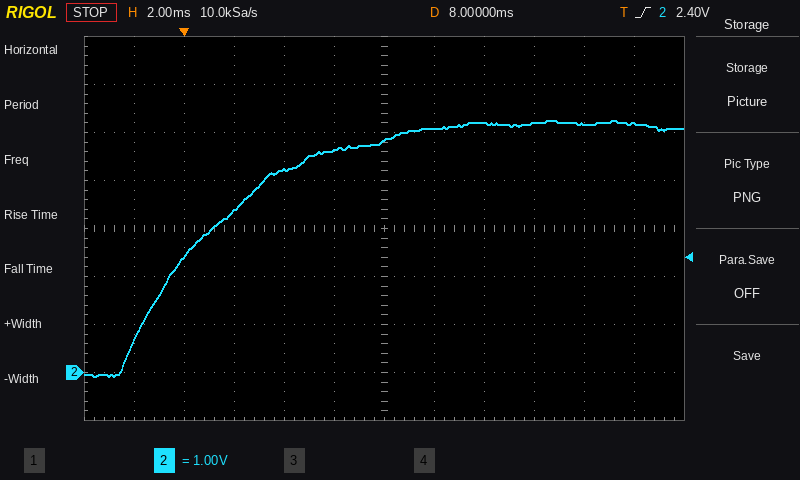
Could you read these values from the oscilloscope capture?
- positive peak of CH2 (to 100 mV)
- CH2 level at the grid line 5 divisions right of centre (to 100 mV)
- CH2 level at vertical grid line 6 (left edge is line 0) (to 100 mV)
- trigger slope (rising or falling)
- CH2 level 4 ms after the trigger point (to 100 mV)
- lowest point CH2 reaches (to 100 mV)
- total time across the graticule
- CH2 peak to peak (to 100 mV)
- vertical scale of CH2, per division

5.2 V
5.2 V
4.8 V
rising
4.2 V
-100 mV
24 ms
5.3 V
1 V
